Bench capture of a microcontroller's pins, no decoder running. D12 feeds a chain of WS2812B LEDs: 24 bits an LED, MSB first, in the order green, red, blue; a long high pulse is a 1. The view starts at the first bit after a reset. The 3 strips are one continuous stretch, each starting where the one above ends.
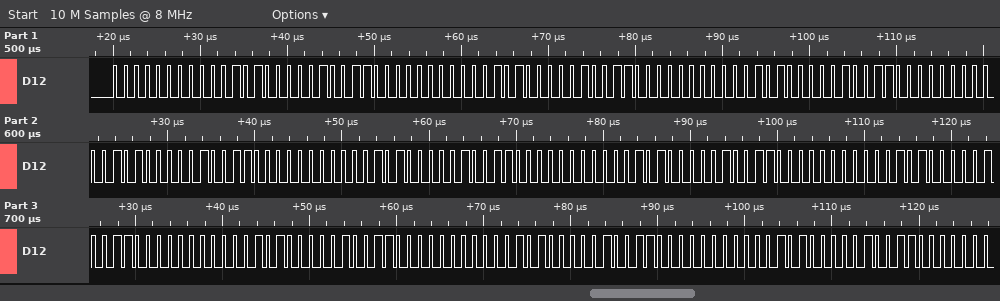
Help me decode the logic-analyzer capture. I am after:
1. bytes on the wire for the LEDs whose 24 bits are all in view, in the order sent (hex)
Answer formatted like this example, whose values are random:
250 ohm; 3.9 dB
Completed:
00 14 13 00 14 13 00 14 13 00 14 13 00 14 13 00 14 13 00 14 13 00 14 13 00 14 13 00 14 13
